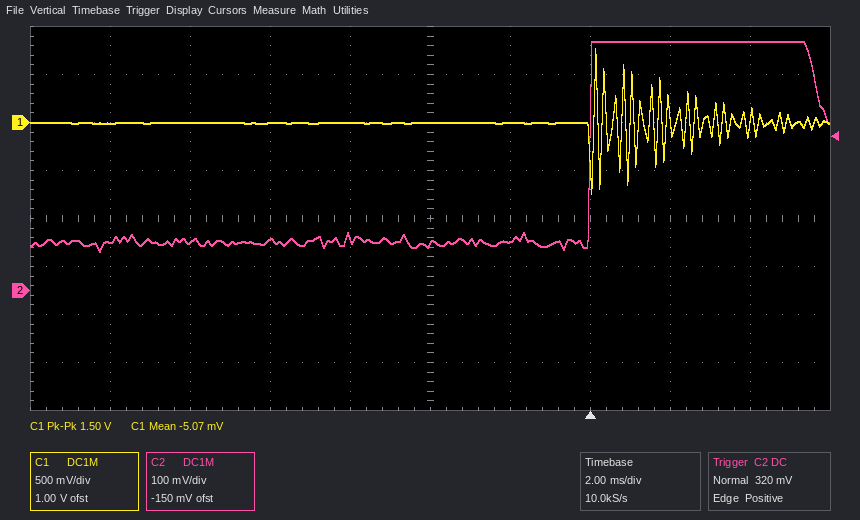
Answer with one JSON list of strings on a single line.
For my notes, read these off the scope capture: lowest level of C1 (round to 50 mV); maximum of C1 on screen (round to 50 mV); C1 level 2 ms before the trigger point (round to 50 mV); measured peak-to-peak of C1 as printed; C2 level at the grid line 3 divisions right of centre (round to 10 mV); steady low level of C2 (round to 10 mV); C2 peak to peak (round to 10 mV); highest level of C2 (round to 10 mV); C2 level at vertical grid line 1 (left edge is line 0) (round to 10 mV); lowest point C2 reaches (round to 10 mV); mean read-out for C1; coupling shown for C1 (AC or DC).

["-750 mV", "750 mV", "0 mV", "1.50 V", "520 mV", "100 mV", "440 mV", "520 mV", "100 mV", "80 mV", "-5.07 mV", "DC"]
